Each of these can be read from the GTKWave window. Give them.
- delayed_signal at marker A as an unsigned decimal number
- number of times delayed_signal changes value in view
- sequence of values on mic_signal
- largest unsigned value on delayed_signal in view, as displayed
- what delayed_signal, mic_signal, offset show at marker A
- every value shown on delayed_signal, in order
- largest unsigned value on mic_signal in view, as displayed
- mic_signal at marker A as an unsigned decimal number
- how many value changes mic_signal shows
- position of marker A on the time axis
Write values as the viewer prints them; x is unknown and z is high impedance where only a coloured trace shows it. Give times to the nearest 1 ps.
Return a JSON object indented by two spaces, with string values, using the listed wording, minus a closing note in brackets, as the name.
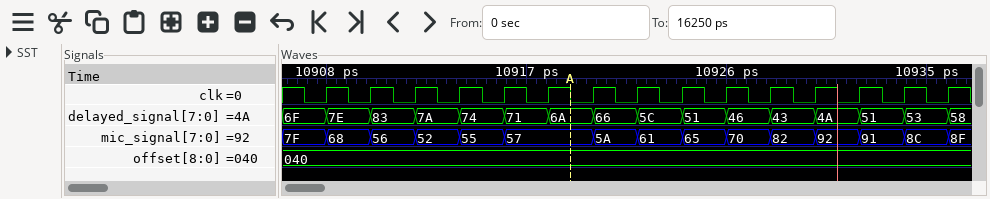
{
  "delayed_signal at marker A as an unsigned decimal number": "106",
  "number of times delayed_signal changes value in view": "15",
  "sequence of values on mic_signal": "7F, 68, 56, 52, 55, 57, 5A, 61, 65, 70, 82, 92, 91, 8C, 8F",
  "largest unsigned value on delayed_signal in view, as displayed": "83",
  "what delayed_signal, mic_signal, offset show at marker A": "delayed_signal=6A, mic_signal=57, offset=040",
  "every value shown on delayed_signal, in order": "6F, 7E, 83, 7A, 74, 71, 6A, 66, 5C, 51, 46, 43, 4A, 51, 53, 58",
  "largest unsigned value on mic_signal in view, as displayed": "92",
  "mic_signal at marker A as an unsigned decimal number": "87",
  "how many value changes mic_signal shows": "14",
  "position of marker A on the time axis": "10919 ps"
}
